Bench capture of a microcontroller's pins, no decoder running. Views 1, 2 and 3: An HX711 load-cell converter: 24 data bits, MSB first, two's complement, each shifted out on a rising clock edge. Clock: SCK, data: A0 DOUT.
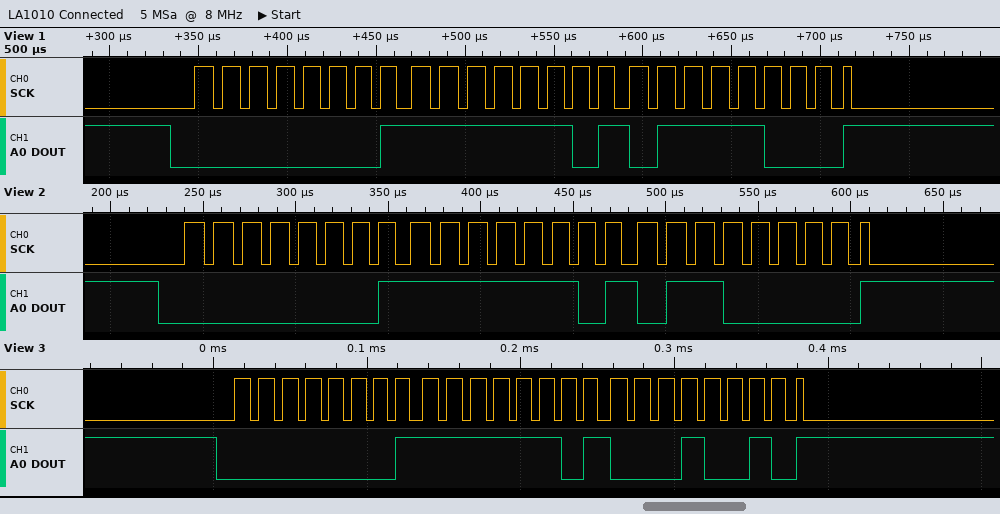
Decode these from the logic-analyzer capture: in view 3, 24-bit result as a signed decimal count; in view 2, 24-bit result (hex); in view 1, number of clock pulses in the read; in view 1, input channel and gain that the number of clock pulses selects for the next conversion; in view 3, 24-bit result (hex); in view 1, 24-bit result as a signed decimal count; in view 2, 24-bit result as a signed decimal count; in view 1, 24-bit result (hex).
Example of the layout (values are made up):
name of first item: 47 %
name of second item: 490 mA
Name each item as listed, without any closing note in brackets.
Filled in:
in view 3, 24-bit result as a signed decimal count: 130322
in view 2, 24-bit result: 0x01FD60
in view 1, number of clock pulses in the read: 25
in view 1, input channel and gain that the number of clock pulses selects for the next conversion: channel A, gain 128
in view 3, 24-bit result: 0x01FD12
in view 1, 24-bit result as a signed decimal count: 130424
in view 2, 24-bit result as a signed decimal count: 130400
in view 1, 24-bit result: 0x01FD78
